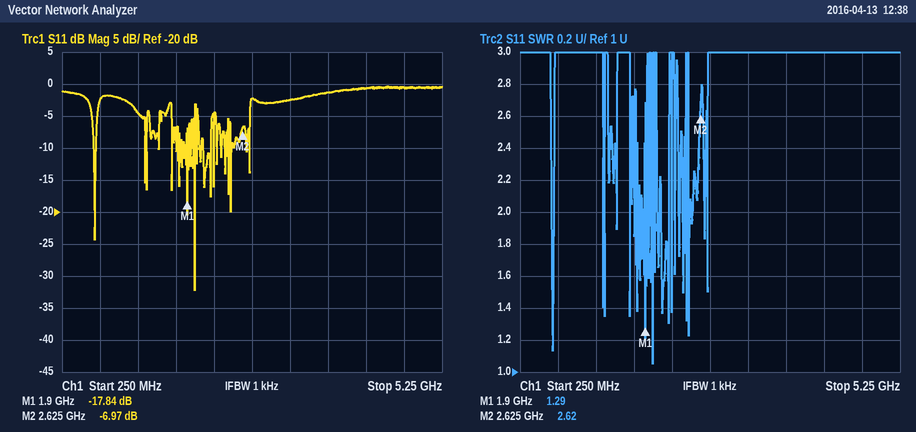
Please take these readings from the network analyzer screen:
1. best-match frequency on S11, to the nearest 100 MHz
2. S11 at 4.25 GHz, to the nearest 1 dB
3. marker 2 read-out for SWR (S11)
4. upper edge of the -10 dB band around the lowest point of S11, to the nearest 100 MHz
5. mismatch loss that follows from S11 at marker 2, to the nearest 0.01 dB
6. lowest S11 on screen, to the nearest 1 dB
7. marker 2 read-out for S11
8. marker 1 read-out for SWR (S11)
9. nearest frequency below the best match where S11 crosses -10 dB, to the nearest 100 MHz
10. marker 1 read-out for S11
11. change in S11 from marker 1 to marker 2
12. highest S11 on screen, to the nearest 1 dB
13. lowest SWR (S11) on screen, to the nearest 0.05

2.0 GHz
-1 dB
2.62
2.0 GHz
0.97 dB
-32 dB
-6.97 dB
1.29
2.0 GHz
-17.84 dB
10.87 dB
0 dB
1.05
